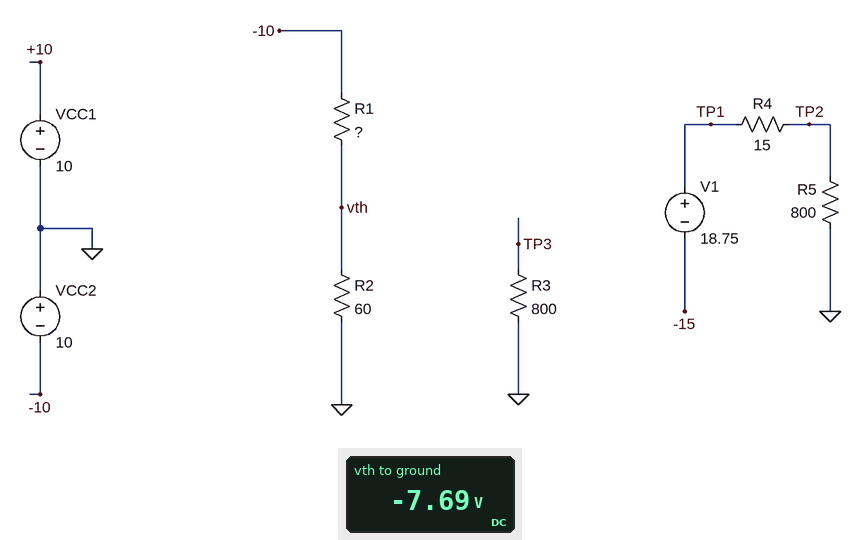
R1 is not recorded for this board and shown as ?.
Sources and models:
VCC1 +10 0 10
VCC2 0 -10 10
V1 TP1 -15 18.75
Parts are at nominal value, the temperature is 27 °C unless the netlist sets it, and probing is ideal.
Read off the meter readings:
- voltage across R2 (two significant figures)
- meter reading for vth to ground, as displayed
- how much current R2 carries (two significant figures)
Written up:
7.7 V
-7.69 V
130 mA
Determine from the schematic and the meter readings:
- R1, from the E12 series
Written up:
18 Ω
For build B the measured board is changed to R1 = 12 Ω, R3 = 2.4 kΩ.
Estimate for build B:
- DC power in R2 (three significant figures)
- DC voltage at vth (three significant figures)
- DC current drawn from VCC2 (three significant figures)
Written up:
1.16 W
-8.33 V
139 mA
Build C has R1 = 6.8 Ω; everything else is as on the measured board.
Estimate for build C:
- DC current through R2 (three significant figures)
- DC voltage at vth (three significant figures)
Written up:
150 mA
-8.98 V
